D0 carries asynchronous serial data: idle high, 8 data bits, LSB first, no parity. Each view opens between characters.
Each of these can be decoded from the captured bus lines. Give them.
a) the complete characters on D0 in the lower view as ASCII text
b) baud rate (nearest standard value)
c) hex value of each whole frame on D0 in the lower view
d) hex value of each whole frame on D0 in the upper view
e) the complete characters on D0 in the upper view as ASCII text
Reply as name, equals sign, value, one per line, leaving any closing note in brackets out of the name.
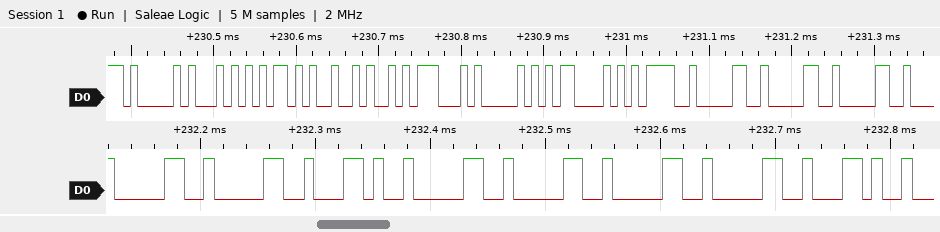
the complete characters on D0 in the lower view as ASCII text = "00,0000,"
baud rate = 115200 baud
hex value of each whole frame on D0 in the lower view = 30, 30, 2C, 30, 30, 30, 30, 2C
hex value of each whole frame on D0 in the upper view = 41, 54, 2B, 4A, 47, 50, 43, 3D, 30, 30, 30
the complete characters on D0 in the upper view as ASCII text = "AT+JGPC=000"
